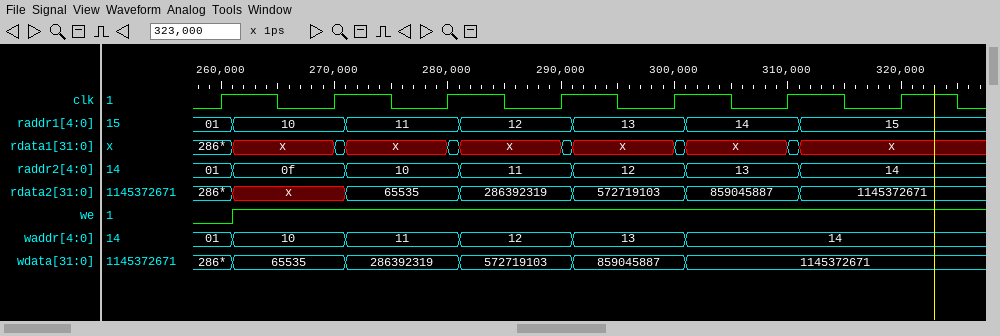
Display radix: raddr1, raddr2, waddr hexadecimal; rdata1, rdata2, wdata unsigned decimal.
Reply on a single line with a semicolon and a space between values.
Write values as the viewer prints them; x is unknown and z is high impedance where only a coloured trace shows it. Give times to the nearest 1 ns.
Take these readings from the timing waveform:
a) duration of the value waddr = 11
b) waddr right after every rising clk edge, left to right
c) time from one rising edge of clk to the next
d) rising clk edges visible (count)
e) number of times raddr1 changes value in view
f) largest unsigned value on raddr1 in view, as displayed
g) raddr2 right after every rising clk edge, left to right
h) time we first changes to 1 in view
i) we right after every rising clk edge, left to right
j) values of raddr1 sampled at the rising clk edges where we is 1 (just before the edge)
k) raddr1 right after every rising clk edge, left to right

10 ns; 01, 10, 11, 12, 13, 14, 14; 10 ns; 7; 6; 15; 01, 0f, 10, 11, 12, 13, 14; 261 ns; 0 1 1 1 1 1 1; 10, 11, 12, 13, 14, 15; 01, 10, 11, 12, 13, 14, 15
